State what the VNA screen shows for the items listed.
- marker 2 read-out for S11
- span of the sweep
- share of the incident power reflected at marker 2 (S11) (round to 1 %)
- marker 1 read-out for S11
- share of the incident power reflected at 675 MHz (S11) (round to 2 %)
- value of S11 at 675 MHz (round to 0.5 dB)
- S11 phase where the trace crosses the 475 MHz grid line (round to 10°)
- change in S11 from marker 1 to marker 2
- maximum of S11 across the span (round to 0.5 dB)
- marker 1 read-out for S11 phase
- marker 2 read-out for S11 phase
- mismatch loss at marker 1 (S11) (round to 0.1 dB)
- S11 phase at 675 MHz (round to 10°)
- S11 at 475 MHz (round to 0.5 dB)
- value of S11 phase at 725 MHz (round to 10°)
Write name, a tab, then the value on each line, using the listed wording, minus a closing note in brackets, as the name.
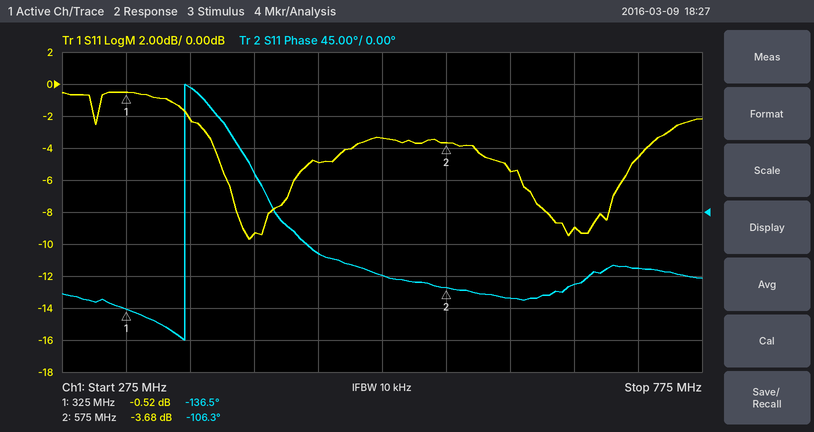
marker 2 read-out for S11	-3.68 dB
span of the sweep	500 MHz
share of the incident power reflected at marker 2 (S11)	43 %
marker 1 read-out for S11	-0.52 dB
share of the incident power reflected at 675 MHz (S11)	12 %
value of S11 at 675 MHz	-9.0 dB
S11 phase where the trace crosses the 475 MHz grid line	-60°
change in S11 from marker 1 to marker 2	-3.16 dB
maximum of S11 across the span	-0.5 dB
marker 1 read-out for S11 phase	-136.5°
marker 2 read-out for S11 phase	-106.3°
mismatch loss at marker 1 (S11)	9.5 dB
S11 phase at 675 MHz	-100°
S11 at 475 MHz	-5.0 dB
value of S11 phase at 725 MHz	-80°
